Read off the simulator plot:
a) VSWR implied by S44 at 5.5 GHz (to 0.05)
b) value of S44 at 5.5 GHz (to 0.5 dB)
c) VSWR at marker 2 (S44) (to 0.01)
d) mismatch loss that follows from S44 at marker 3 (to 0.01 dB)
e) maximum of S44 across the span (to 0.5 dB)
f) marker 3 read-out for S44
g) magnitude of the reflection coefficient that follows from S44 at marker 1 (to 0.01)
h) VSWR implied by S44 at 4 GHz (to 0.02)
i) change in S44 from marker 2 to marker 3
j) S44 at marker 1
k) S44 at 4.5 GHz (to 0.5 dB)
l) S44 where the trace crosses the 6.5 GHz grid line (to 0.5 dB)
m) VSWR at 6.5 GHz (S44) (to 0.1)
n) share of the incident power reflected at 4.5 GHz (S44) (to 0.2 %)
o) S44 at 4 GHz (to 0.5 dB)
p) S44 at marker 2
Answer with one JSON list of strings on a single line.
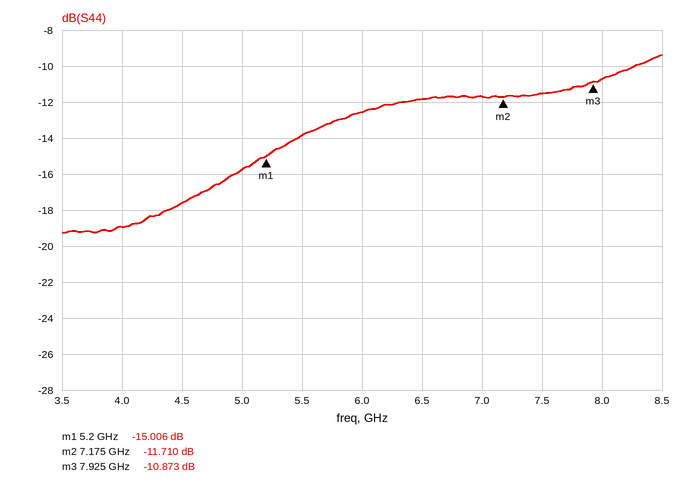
["1.50", "-14.0 dB", "1.70", "0.37 dB", "-9.5 dB", "-10.873 dB", "0.18", "1.26", "0.837 dB", "-15.006 dB", "-17.5 dB", "-12.0 dB", "1.7", "1.8 %", "-19.0 dB", "-11.710 dB"]
